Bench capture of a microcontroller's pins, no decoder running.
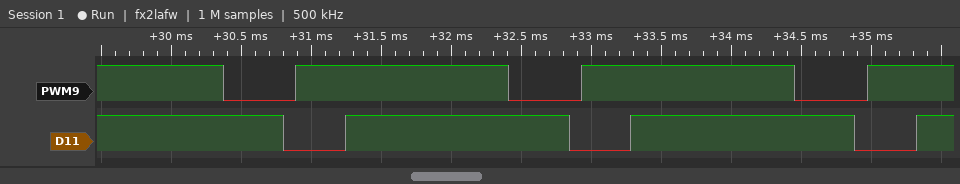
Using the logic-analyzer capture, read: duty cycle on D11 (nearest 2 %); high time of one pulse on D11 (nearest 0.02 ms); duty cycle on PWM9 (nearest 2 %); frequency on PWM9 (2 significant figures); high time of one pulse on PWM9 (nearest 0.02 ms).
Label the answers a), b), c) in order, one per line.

a) 78 %
b) 1.60 ms
c) 74 %
d) 490 Hz
e) 1.52 ms
